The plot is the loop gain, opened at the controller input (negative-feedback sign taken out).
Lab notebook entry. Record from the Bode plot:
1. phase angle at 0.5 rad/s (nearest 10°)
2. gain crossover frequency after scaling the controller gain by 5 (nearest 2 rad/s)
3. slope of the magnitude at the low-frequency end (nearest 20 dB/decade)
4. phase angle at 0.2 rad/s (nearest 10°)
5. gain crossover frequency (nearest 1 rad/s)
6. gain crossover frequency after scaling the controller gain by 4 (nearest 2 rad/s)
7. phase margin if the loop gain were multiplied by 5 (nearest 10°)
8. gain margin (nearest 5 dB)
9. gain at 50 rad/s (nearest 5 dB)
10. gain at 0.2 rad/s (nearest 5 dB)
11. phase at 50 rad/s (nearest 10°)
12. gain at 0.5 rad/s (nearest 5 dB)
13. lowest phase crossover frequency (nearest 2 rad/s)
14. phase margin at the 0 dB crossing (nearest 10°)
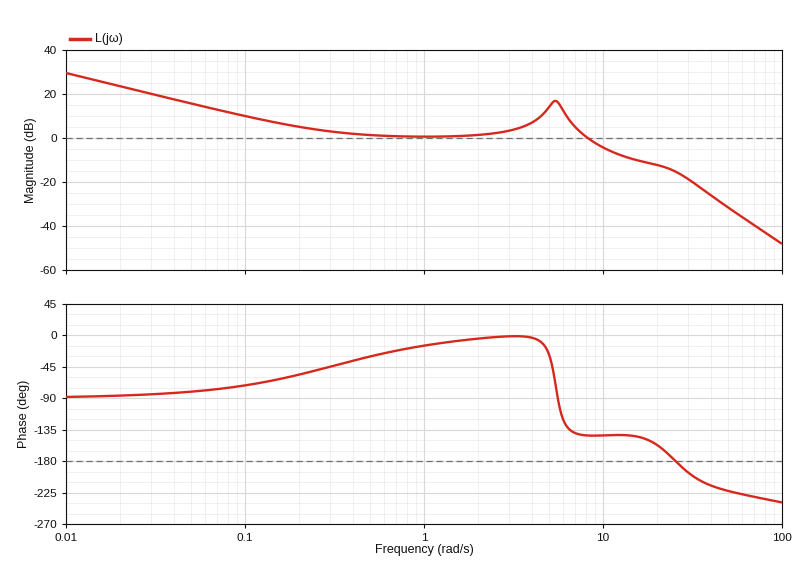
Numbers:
-30°
24 rad/s
-20 dB/decade
-60°
8 rad/s
20 rad/s
10°
15 dB
-30 dB
5 dB
-220°
0 dB
26 rad/s
40°
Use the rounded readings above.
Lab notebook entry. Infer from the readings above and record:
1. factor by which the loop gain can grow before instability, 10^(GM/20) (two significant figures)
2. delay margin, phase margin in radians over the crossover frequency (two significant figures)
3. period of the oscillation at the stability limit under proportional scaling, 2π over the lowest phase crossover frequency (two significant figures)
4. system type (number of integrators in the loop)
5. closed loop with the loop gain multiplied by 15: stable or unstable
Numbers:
5.6
0.087 s
0.24 s
1
unstable
